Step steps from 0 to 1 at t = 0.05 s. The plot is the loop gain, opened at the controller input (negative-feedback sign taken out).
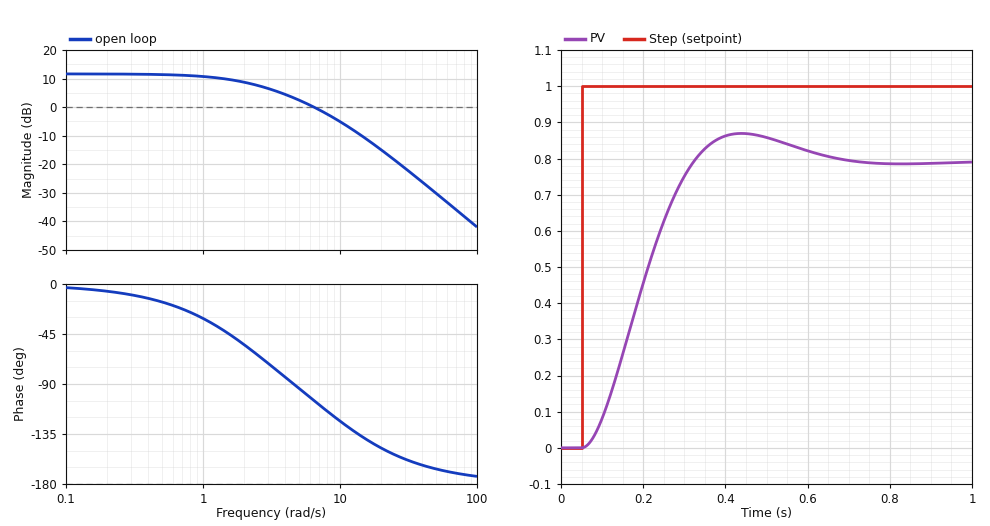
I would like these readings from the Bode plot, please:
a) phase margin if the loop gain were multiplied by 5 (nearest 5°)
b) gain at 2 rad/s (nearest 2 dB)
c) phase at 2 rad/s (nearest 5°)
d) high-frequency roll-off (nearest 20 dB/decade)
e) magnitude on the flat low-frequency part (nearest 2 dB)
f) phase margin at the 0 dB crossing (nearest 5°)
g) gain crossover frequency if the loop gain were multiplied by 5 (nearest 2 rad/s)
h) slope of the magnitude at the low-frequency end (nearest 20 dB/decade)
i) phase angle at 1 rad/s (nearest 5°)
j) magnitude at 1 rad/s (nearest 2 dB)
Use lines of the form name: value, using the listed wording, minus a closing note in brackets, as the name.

phase margin if the loop gain were multiplied by 5: 35°
gain at 2 rad/s: 8 dB
phase at 2 rad/s: -55°
high-frequency roll-off: -40 dB/decade
magnitude on the flat low-frequency part: 12 dB
phase margin at the 0 dB crossing: 75°
gain crossover frequency if the loop gain were multiplied by 5: 18 rad/s
slope of the magnitude at the low-frequency end: 0 dB/decade
phase angle at 1 rad/s: -30°
magnitude at 1 rad/s: 10 dB
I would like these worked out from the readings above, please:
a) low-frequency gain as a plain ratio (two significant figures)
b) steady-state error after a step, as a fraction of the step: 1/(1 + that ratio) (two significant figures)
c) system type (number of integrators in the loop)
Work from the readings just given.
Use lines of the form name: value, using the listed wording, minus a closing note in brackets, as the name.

low-frequency gain as a plain ratio: 4.0
steady-state error after a step, as a fraction of the step: 1/(1 + that ratio): 0.20
system type: 0
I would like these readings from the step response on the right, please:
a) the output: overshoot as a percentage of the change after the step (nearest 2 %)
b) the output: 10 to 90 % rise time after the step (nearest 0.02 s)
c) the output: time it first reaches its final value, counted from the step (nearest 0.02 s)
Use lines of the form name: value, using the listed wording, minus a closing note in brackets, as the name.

the output: overshoot as a percentage of the change after the step: 10 %
the output: 10 to 90 % rise time after the step: 0.18 s
the output: time it first reaches its final value, counted from the step: 0.28 s
